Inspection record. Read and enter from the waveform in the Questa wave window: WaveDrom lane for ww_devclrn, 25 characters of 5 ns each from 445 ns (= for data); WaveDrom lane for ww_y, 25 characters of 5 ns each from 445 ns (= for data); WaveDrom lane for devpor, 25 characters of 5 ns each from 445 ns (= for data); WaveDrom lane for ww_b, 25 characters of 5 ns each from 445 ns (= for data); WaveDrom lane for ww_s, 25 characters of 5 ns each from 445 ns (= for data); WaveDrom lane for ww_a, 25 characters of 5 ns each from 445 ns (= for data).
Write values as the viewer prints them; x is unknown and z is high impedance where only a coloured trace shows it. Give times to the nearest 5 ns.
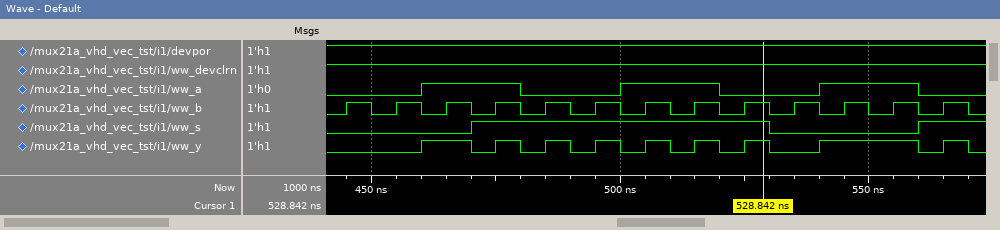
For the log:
{name: 'ww_devclrn', wave: '1........................'}
{name: 'ww_y', wave: '0..1.0101010101010.1...01'}
{name: 'devpor', wave: '1........................'}
{name: 'ww_b', wave: '1010101010101010101010101'}
{name: 'ww_s', wave: '0....1...........0.....1.'}
{name: 'ww_a', wave: '0..1...0...1...0...1...0.'}
